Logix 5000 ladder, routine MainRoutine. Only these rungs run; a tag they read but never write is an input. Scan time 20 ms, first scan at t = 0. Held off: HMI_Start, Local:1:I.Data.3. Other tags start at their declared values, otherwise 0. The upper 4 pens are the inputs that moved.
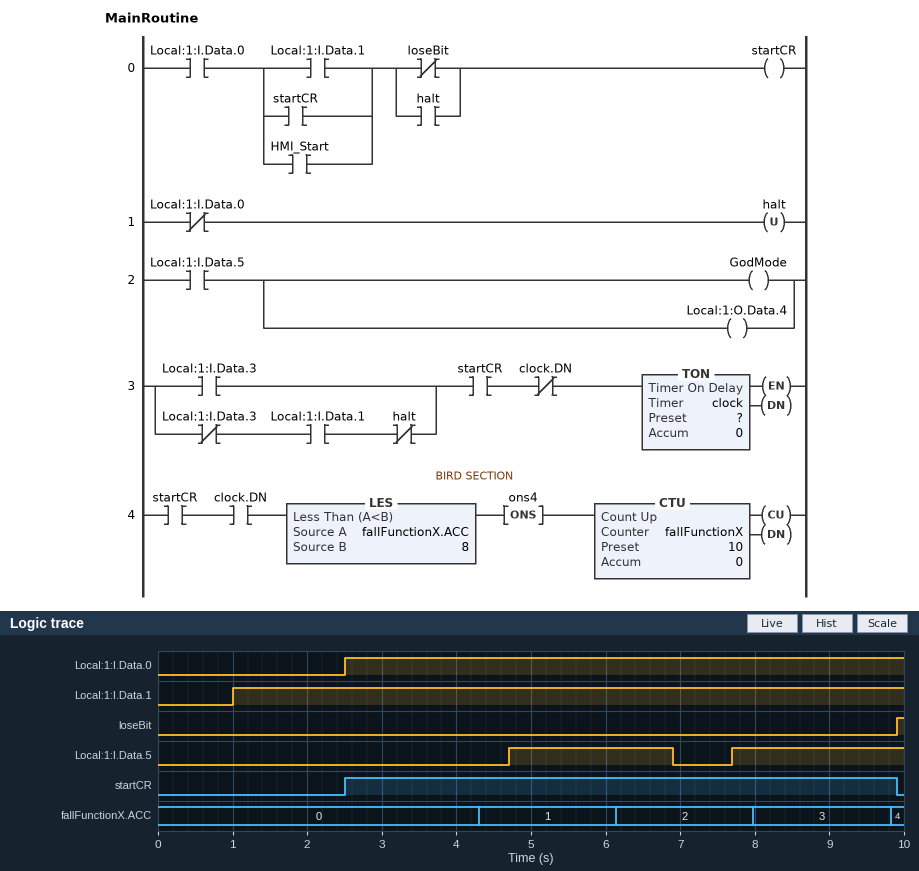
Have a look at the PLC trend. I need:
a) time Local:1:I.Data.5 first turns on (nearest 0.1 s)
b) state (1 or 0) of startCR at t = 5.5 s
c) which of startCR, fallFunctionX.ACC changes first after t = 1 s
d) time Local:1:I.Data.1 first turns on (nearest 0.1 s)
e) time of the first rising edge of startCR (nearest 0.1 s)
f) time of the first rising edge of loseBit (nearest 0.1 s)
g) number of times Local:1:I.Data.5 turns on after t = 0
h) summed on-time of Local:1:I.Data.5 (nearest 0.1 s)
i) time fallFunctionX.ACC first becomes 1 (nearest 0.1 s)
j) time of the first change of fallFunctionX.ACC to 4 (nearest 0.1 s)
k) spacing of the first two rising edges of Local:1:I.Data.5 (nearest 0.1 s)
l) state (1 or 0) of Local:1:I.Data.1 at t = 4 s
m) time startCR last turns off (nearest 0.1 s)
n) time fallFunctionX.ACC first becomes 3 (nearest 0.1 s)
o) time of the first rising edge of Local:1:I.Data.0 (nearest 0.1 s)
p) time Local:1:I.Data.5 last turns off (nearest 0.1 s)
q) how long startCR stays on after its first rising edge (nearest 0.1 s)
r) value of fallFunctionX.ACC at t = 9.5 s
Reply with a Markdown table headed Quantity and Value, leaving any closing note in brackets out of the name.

| Quantity | Value |
|---|---|
| time Local:1:I.Data.5 first turns on | 4.7 s |
| state (1 or 0) of startCR at t = 5.5 s | 1 |
| which of startCR, fallFunctionX.ACC changes first after t = 1 s | startCR |
| time Local:1:I.Data.1 first turns on | 1.0 s |
| time of the first rising edge of startCR | 2.5 s |
| time of the first rising edge of loseBit | 9.9 s |
| number of times Local:1:I.Data.5 turns on after t = 0 | 2 |
| summed on-time of Local:1:I.Data.5 | 4.5 s |
| time fallFunctionX.ACC first becomes 1 | 4.3 s |
| time of the first change of fallFunctionX.ACC to 4 | 9.8 s |
| spacing of the first two rising edges of Local:1:I.Data.5 | 3.0 s |
| state (1 or 0) of Local:1:I.Data.1 at t = 4 s | 1 |
| time startCR last turns off | 9.9 s |
| time fallFunctionX.ACC first becomes 3 | 8.0 s |
| time of the first rising edge of Local:1:I.Data.0 | 2.5 s |
| time Local:1:I.Data.5 last turns off | 6.9 s |
| how long startCR stays on after its first rising edge | 7.4 s |
| value of fallFunctionX.ACC at t = 9.5 s | 3 |
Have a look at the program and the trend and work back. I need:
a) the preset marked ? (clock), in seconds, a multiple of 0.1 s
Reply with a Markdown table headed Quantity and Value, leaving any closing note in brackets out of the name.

| Quantity | Value |
|---|---|
| the preset marked ? (clock), in seconds, a multiple of 0.1 s | 1.8 s |
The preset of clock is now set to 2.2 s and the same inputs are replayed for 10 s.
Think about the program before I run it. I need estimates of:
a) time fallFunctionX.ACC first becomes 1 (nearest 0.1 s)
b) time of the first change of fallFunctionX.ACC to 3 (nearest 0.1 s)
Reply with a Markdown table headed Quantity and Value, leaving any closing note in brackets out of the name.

| Quantity | Value |
|---|---|
| time fallFunctionX.ACC first becomes 1 | 4.7 s |
| time of the first change of fallFunctionX.ACC to 3 | 9.2 s |
